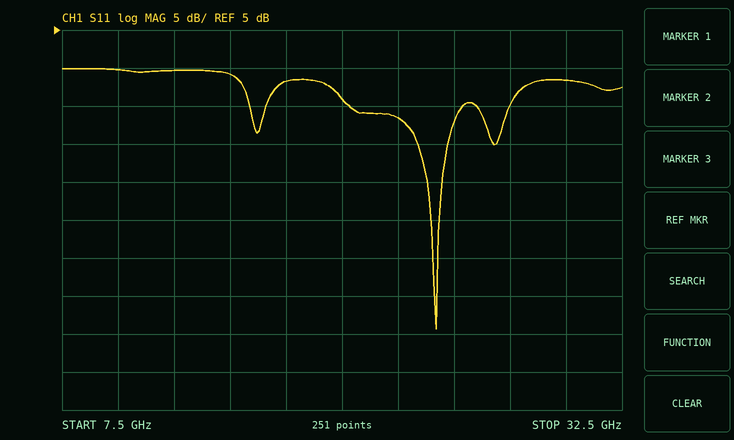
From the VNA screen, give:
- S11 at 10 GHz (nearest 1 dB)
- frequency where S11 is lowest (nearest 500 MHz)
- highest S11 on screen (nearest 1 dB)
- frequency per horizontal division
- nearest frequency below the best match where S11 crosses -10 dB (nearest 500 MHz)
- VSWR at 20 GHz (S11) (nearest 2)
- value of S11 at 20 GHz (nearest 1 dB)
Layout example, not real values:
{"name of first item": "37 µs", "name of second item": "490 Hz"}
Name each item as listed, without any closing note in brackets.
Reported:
{"S11 at 10 GHz": "0 dB", "frequency where S11 is lowest": "24.0 GHz", "highest S11 on screen": "0 dB", "frequency per horizontal division": "2.5 GHz", "nearest frequency below the best match where S11 crosses -10 dB": "23.5 GHz", "VSWR at 20 GHz (S11)": "4", "value of S11 at 20 GHz": "-4 dB"}
